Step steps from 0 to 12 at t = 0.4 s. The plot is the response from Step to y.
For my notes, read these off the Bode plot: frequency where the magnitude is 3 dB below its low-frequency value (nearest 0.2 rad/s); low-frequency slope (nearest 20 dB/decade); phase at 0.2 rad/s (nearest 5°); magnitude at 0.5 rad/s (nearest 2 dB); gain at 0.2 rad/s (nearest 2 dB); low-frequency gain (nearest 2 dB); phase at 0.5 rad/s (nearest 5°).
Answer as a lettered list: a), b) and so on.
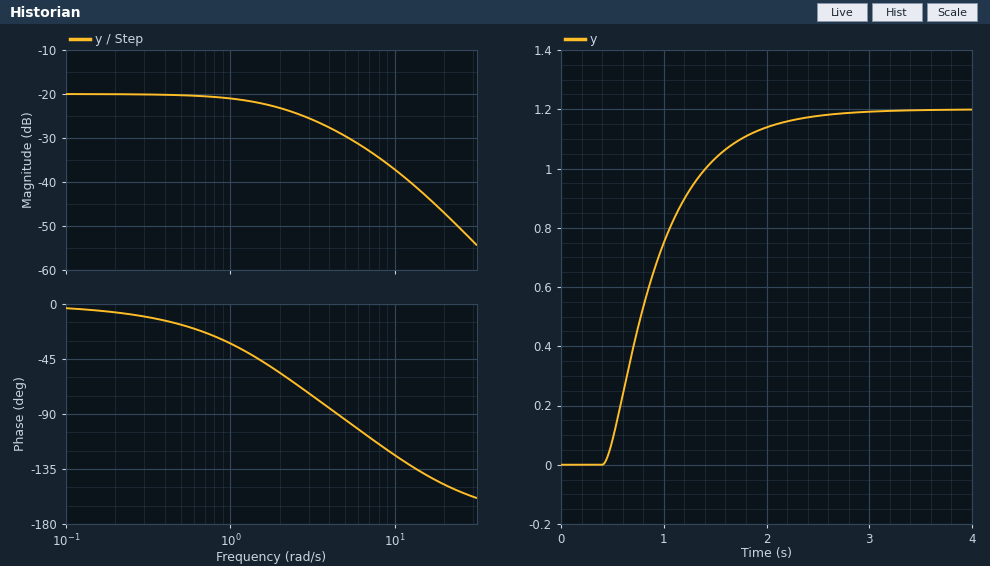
a) 2.0 rad/s
b) 0 dB/decade
c) -5°
d) -20 dB
e) -20 dB
f) -20 dB
g) -15°
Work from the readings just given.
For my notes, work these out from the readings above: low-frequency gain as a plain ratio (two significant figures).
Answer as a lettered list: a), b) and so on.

a) 0.10
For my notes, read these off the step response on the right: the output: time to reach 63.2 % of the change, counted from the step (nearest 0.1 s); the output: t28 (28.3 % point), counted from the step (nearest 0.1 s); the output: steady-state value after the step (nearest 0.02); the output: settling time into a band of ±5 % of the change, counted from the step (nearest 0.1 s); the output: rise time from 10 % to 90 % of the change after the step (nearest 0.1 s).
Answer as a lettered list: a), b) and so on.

a) 0.6 s
b) 0.3 s
c) 1.20
d) 1.6 s
e) 1.1 s
